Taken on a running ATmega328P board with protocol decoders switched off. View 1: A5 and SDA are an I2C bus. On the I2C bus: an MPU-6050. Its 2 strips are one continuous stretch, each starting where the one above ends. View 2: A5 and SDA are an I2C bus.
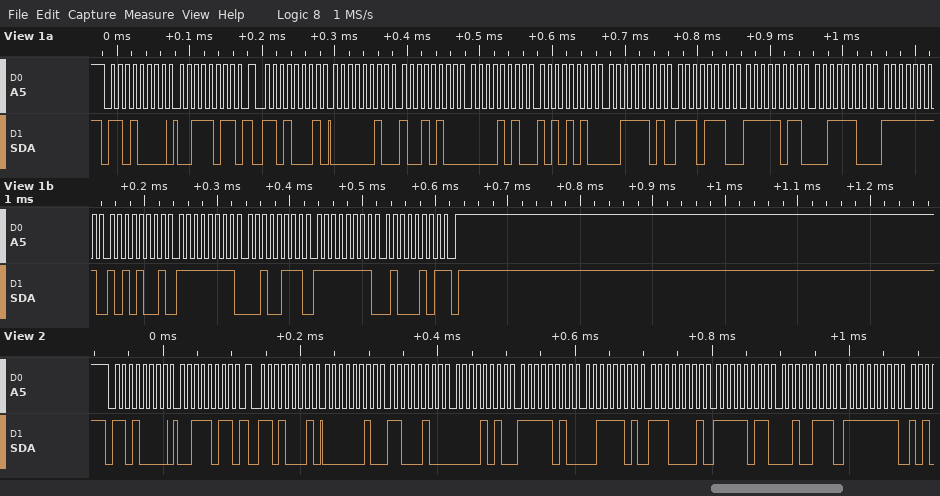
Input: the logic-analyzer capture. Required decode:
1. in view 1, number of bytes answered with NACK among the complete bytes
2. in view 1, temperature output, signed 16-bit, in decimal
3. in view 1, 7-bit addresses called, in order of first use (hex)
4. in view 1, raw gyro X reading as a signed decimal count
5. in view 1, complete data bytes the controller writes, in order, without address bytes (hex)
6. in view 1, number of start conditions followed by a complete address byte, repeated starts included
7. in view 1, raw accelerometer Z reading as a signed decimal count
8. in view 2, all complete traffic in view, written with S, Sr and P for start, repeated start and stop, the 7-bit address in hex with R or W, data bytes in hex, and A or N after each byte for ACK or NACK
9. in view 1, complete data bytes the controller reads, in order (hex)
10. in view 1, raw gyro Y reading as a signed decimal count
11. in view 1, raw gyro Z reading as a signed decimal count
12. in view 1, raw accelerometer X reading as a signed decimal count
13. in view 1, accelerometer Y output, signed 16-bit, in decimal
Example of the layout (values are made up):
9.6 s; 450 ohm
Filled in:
1; -1220; 0x68; -87; 3B; 2; 15854; S 68W A 3B A Sr 68R A 02 A C4 A 0A A FA A 3D A E1 A FB A 27 A FF A; 02 94 0A AA 3D EE FB 3C FF A9 FF 27 FF 45; -217; -187; 660; 2730
